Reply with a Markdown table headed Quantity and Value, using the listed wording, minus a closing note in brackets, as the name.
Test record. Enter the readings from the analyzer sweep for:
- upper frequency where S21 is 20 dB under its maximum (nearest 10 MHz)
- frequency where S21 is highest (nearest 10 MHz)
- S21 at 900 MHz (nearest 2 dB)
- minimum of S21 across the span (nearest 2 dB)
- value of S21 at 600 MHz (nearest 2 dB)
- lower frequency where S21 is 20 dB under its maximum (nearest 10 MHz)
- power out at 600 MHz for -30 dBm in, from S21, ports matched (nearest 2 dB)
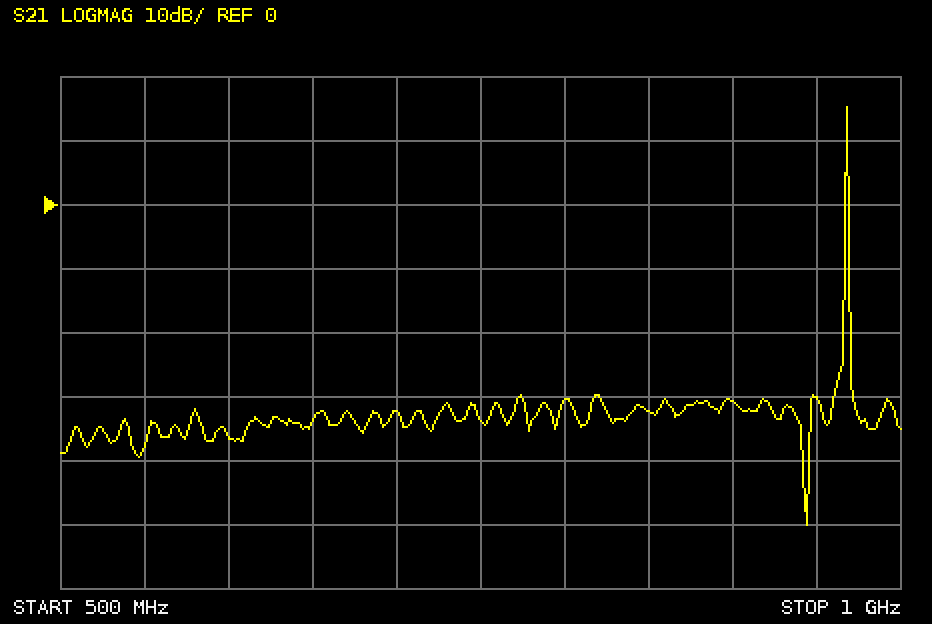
| Quantity | Value |
|---|---|
| upper frequency where S21 is 20 dB under its maximum | 970 MHz |
| frequency where S21 is highest | 970 MHz |
| S21 at 900 MHz | -30 dB |
| minimum of S21 across the span | -50 dB |
| value of S21 at 600 MHz | -36 dB |
| lower frequency where S21 is 20 dB under its maximum | 970 MHz |
| power out at 600 MHz for -30 dBm in, from S21, ports matched | -66 dBm |
